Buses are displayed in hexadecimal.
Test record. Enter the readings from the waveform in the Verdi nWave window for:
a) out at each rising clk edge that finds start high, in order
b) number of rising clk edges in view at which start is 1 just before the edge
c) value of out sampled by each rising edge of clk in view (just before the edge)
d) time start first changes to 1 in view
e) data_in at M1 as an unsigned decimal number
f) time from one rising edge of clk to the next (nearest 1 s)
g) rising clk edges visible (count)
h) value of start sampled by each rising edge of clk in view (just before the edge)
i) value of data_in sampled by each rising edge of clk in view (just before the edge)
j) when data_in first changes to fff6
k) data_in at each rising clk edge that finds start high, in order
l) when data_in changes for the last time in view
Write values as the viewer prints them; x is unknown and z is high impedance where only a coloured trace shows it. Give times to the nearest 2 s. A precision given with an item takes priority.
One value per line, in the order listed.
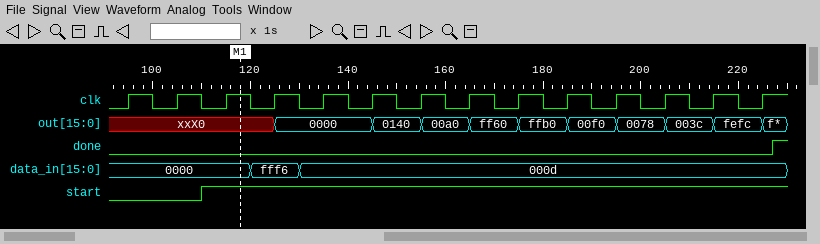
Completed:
xxX0, xxX0, 0000, 0000, 0140, 00a0, ff60, ffb0, 00f0, 0078, 003c, fefc
12
xxX0, xxX0, xxX0, xxX0, 0000, 0000, 0140, 00a0, ff60, ffb0, 00f0, 0078, 003c, fefc
110 s
0
10 s
14
0 0 1 1 1 1 1 1 1 1 1 1 1 1
0000, 0000, 0000, fff6, 000d, 000d, 000d, 000d, 000d, 000d, 000d, 000d, 000d, 000d
120 s
0000, fff6, 000d, 000d, 000d, 000d, 000d, 000d, 000d, 000d, 000d, 000d
130 s
